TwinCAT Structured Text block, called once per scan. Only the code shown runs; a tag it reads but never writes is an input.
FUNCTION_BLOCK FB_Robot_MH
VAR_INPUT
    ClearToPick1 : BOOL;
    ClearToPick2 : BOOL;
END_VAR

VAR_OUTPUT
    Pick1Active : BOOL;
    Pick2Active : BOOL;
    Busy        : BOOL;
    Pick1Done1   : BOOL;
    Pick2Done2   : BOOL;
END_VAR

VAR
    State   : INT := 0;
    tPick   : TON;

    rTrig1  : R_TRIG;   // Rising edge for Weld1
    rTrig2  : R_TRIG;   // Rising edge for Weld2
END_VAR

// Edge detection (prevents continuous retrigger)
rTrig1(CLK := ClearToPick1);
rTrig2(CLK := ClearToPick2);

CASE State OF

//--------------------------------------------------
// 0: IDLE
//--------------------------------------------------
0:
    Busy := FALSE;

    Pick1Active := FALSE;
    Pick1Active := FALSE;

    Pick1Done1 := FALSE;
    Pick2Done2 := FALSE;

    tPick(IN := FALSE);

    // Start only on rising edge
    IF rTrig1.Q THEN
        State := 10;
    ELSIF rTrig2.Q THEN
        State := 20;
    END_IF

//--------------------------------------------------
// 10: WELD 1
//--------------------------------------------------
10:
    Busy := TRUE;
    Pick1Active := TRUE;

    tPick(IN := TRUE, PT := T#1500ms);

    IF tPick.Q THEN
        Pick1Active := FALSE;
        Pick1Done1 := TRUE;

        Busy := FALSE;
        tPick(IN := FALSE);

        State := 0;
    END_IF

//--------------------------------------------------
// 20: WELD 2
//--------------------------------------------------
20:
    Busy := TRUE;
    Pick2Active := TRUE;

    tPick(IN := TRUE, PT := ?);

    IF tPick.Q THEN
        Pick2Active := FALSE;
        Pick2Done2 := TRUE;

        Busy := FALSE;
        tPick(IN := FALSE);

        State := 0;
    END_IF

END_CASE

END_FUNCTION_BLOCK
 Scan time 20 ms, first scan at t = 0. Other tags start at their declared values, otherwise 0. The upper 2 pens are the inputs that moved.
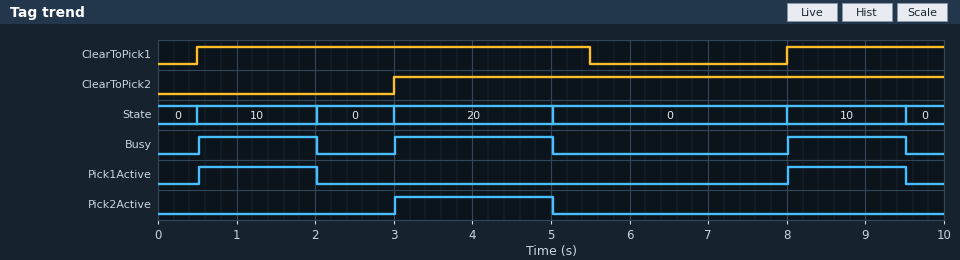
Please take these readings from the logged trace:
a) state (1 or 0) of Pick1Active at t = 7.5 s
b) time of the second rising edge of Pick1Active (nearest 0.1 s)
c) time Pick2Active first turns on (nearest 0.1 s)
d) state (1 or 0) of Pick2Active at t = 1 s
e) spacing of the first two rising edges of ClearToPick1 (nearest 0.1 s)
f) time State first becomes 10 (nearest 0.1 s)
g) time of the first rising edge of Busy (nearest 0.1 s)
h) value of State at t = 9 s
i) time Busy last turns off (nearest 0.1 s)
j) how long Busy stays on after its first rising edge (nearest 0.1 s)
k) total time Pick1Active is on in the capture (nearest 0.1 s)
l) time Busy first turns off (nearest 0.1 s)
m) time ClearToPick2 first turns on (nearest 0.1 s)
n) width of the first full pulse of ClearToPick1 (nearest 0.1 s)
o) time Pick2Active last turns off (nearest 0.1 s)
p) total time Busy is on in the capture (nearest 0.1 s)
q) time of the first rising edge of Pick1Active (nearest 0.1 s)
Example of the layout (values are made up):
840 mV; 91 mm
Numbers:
0; 8.0 s; 3.0 s; 0; 7.5 s; 0.5 s; 0.5 s; 10; 9.5 s; 1.5 s; 3.0 s; 2.0 s; 3.0 s; 5.0 s; 5.0 s; 5.0 s; 0.5 s
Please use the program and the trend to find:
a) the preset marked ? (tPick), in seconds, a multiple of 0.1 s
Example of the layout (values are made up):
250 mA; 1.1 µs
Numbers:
2.0 s
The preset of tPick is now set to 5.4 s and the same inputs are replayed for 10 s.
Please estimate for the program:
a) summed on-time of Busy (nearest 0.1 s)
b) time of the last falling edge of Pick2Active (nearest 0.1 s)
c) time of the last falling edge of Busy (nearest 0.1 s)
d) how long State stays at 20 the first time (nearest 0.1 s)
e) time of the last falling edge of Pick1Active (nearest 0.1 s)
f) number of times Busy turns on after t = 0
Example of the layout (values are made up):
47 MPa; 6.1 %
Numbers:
6.9 s; 8.4 s; 8.4 s; 5.4 s; 2.0 s; 2
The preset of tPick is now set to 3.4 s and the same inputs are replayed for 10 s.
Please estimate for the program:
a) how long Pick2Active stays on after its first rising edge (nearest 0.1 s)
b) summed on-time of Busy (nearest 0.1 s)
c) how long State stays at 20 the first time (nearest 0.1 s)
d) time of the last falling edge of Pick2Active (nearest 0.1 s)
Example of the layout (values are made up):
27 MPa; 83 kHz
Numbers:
3.4 s; 6.4 s; 3.4 s; 6.4 s
